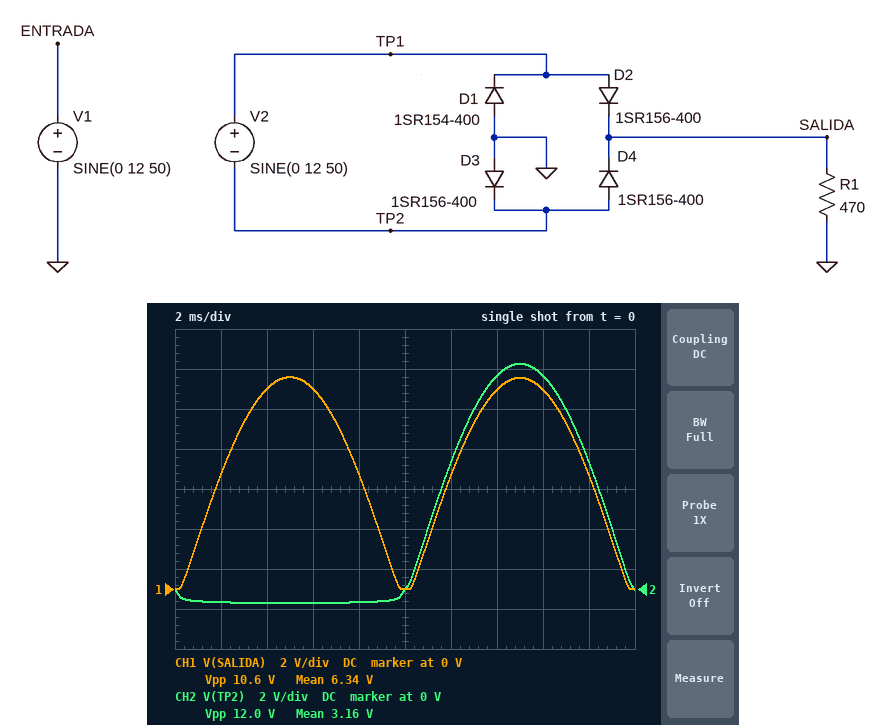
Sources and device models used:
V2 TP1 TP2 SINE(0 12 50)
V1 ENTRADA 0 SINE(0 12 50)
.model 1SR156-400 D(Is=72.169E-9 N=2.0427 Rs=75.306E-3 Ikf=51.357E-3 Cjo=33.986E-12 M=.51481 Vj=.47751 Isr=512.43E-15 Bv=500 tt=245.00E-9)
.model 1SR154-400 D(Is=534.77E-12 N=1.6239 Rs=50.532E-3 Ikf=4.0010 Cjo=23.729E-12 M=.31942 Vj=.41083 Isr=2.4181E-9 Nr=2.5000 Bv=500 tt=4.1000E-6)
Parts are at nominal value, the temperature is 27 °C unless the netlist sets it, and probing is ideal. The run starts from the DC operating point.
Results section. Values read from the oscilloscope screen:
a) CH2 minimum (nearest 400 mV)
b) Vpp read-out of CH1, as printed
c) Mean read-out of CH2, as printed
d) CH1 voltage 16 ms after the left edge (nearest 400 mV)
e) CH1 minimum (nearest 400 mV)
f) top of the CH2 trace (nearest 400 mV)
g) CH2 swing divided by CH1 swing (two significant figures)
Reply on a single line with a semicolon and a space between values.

-800 mV; 10.6 V; 3.16 V; 10.0 V; 0 V; 11.2 V; 1.1
